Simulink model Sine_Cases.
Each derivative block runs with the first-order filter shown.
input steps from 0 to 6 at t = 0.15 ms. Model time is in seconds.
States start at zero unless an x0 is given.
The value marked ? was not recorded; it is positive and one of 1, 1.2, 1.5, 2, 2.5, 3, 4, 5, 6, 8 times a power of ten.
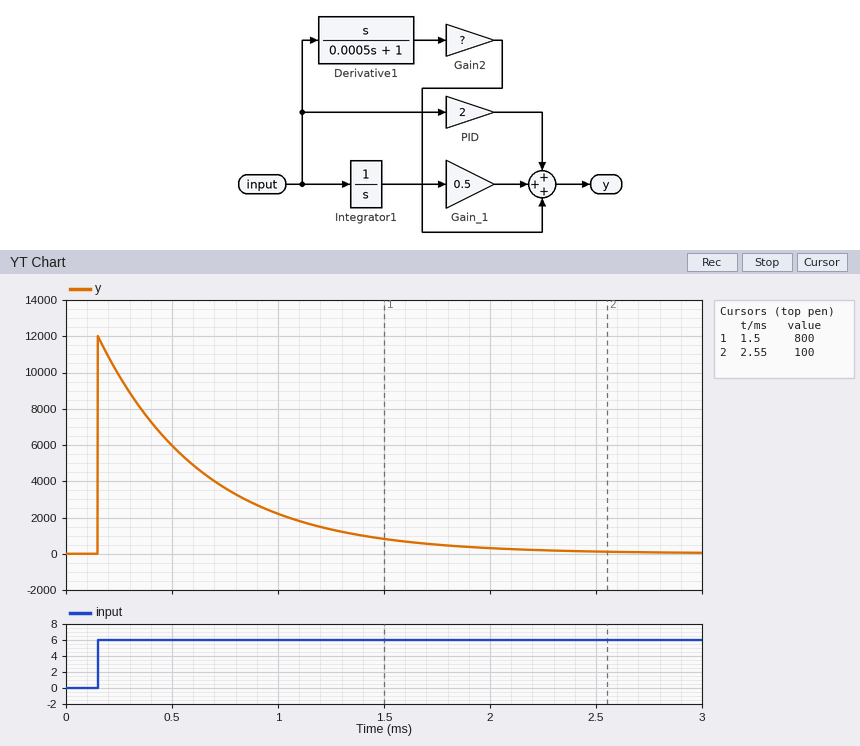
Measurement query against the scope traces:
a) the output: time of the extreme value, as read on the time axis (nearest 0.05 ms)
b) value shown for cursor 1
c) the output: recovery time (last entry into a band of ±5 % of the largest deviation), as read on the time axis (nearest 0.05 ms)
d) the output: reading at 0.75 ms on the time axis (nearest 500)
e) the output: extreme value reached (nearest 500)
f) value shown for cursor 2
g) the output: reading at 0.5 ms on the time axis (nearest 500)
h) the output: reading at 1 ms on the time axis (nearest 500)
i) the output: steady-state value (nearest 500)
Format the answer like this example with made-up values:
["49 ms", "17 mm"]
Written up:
["0.15 ms", "800", "1.65 ms", "3500", "12000", "100", "6000", "2000", "0"]
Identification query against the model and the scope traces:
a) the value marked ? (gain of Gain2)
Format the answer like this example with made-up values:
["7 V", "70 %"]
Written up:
["1"]
